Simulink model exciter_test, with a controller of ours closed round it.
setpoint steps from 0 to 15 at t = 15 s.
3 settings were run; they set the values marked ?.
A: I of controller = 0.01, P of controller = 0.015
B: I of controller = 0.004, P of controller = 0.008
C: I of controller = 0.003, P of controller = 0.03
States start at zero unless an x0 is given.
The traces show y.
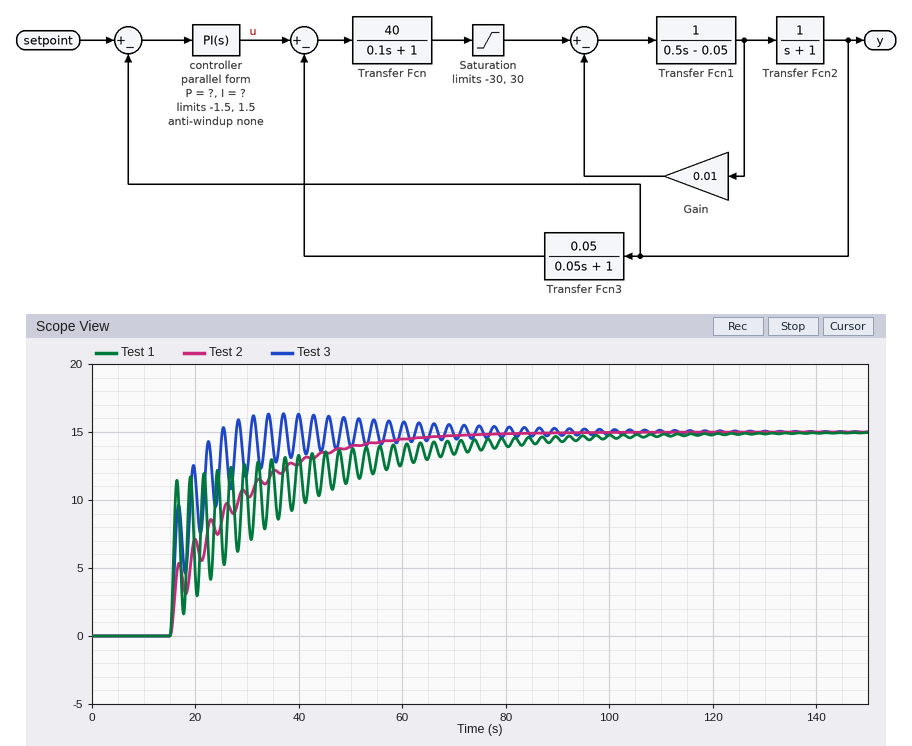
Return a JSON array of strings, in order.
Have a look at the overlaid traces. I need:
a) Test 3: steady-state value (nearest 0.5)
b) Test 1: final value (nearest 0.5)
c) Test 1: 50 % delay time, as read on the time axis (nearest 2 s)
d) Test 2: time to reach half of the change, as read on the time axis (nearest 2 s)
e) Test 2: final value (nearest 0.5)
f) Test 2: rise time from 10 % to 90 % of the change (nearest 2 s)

["15.0", "15.0", "16 s", "22 s", "15.0", "28 s"]
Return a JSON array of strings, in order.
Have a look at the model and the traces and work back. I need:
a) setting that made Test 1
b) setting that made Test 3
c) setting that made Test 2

["C", "A", "B"]
